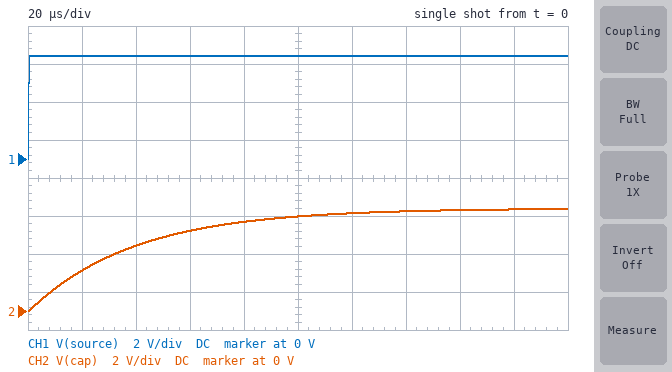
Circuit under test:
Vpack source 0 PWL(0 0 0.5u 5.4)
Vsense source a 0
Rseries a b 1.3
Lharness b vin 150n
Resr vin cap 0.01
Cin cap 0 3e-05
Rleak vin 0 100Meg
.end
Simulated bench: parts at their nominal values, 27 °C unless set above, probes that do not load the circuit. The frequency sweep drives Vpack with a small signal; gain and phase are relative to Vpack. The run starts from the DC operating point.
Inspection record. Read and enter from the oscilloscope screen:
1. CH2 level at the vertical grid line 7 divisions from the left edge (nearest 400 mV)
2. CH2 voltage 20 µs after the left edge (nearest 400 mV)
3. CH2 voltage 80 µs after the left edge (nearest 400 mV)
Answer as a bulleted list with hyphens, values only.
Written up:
- 5.2 V
- 2.0 V
- 4.8 V
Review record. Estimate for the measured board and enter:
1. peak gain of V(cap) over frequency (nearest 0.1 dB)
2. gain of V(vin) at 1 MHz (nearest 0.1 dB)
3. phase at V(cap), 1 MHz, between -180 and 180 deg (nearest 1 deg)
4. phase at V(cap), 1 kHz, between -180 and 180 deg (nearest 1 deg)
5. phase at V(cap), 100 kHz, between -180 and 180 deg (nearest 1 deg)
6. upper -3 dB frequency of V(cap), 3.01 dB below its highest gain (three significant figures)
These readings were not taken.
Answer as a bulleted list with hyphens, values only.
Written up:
- 0 dB
- -43.1 dB
- -126 deg
- -14 deg
- -92 deg
- 4.06 kHz
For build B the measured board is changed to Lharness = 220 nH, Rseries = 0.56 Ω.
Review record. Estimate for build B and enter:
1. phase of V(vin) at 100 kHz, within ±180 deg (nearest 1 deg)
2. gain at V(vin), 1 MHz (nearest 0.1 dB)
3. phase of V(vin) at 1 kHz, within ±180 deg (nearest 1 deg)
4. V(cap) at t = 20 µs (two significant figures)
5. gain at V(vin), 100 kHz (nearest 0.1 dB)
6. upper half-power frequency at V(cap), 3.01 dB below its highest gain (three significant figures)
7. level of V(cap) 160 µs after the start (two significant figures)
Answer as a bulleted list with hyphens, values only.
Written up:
- -88 deg
- -42.4 dB
- -6 deg
- 3.7 V
- -20.6 dB
- 9.52 kHz
- 5.4 V
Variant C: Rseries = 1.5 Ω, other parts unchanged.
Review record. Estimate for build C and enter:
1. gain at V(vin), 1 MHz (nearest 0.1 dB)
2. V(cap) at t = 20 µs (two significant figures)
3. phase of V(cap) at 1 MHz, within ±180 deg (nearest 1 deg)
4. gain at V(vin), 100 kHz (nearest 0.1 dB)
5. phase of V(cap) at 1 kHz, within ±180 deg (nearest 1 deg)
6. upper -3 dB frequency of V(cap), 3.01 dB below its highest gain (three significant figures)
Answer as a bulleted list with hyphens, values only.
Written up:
- -43.9 dB
- 1.9 V
- -122 deg
- -28.9 dB
- -16 deg
- 3.52 kHz
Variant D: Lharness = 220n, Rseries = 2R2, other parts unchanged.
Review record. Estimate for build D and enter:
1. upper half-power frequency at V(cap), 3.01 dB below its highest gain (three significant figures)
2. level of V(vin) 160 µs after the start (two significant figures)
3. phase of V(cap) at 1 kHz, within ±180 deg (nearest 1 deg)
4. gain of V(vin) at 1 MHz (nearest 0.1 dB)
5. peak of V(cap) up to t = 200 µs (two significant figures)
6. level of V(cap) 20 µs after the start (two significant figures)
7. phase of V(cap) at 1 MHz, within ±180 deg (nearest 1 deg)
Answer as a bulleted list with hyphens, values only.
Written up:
- 2.40 kHz
- 4.9 V
- -23 deg
- -47.2 dB
- 5.1 V
- 1.4 V
- -122 deg
